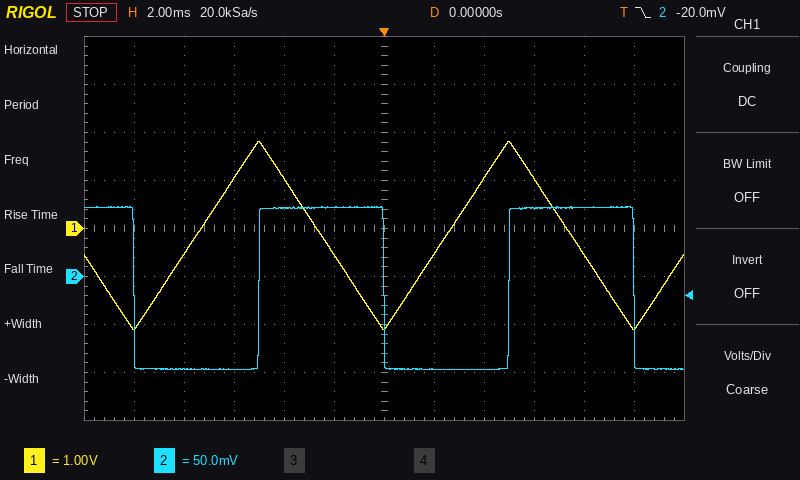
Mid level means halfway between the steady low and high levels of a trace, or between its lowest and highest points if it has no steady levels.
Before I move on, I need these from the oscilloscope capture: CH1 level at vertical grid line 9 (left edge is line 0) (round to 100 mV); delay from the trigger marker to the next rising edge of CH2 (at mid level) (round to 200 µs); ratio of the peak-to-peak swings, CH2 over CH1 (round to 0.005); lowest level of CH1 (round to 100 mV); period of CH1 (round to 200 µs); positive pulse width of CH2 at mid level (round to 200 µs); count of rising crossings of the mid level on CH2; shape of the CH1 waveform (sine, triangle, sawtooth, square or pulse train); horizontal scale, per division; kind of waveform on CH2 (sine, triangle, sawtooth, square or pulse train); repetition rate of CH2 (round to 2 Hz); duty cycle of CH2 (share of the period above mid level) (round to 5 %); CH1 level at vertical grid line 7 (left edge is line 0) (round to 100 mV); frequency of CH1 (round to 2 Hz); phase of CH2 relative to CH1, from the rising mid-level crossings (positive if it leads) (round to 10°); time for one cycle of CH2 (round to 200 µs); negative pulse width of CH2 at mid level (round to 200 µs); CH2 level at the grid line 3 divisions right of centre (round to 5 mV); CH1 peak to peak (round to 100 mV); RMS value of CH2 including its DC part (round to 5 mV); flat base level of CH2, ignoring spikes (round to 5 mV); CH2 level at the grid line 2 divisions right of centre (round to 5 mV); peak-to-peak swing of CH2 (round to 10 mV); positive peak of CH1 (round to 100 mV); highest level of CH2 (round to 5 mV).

1.0 V
5.0 ms
0.045
-2.1 V
10.0 ms
5.0 ms
2
triangle
2 ms
square
100 Hz
50 %
-500 mV
100 Hz
-90°
10.0 ms
5.0 ms
70 mV
3.9 V
85 mV
-95 mV
-95 mV
170 mV
1.8 V
75 mV
